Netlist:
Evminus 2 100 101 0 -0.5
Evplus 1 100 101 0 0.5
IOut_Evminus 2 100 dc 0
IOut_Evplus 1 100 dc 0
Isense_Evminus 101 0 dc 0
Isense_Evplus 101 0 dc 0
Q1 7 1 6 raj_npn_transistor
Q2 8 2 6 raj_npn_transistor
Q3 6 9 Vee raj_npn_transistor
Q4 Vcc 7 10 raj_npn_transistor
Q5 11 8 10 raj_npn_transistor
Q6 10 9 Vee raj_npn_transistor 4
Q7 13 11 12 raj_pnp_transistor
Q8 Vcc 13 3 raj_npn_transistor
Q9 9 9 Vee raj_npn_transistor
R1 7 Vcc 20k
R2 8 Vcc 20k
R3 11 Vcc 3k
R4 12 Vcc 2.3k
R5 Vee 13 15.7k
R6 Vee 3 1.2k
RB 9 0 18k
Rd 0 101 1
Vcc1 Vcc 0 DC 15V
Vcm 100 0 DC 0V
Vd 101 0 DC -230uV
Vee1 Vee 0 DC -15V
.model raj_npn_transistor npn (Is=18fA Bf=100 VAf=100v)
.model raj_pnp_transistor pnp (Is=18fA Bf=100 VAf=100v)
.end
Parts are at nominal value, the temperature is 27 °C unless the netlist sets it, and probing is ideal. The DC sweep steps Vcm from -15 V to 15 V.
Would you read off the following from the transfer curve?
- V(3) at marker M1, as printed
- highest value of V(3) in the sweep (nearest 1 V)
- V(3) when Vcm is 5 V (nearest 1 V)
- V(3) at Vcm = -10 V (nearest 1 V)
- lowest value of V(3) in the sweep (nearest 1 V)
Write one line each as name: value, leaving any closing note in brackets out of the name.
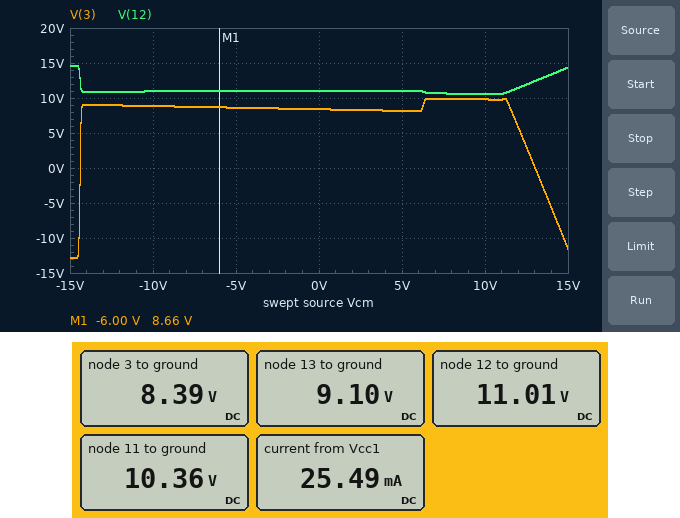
V(3) at marker M1, as printed: 8.66 V
highest value of V(3) in the sweep: 10 V
V(3) when Vcm is 5 V: 8 V
V(3) at Vcm = -10 V: 9 V
lowest value of V(3) in the sweep: -13 V
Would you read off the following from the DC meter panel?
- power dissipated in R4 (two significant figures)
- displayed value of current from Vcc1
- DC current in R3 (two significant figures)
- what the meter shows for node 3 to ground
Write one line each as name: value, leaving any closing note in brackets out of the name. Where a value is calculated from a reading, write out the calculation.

power dissipated in R4: (15 V - 11.01 V)^2 / 2.3 kΩ = 6.9 mW
displayed value of current from Vcc1: 25.49 mA
DC current in R3: (15 V - 10.36 V) / 3 kΩ = 1.5 mA
what the meter shows for node 3 to ground: 8.39 V
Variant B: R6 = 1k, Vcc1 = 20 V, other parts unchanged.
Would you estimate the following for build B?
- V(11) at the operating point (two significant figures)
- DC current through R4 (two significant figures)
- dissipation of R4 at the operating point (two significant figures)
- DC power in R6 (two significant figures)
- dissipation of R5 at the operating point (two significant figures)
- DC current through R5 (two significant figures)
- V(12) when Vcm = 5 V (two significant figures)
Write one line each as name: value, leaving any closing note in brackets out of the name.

V(11) at the operating point: 15 V
DC current through R4: 1.8 mA
dissipation of R4 at the operating point: 7.7 mW
DC power in R6: 590 mW
dissipation of R5 at the operating point: 40 mW
DC current through R5: 1.6 mA
V(12) when Vcm = 5 V: 16 V
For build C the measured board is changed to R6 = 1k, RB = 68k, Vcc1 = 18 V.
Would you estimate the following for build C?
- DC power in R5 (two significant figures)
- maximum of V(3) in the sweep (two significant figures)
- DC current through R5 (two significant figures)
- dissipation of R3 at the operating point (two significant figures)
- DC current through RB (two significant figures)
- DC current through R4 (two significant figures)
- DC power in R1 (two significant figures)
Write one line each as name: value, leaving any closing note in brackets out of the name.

DC power in R5: 1.5 mW
maximum of V(3) in the sweep: -11 V
DC current through R5: 310 µA
dissipation of R3 at the operating point: 650 µW
DC current through RB: 210 µA
DC current through R4: 340 µA
DC power in R1: 280 µW
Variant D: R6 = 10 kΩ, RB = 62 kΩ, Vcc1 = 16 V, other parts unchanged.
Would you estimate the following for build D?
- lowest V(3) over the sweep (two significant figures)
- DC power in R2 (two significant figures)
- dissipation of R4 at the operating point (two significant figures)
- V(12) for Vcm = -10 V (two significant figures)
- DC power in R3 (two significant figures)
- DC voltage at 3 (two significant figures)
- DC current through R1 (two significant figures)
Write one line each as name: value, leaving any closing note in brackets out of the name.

lowest V(3) over the sweep: -15 V
DC power in R2: 330 µW
dissipation of R4 at the operating point: 340 µW
V(12) for Vcm = -10 V: 15 V
DC power in R3: 750 µW
DC voltage at 3: -9.7 V
DC current through R1: 130 µA
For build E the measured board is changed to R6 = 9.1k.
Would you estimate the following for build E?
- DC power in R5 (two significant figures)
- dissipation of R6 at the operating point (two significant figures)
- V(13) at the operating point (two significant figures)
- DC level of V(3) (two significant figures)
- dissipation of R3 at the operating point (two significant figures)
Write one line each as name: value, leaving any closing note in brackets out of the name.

DC power in R5: 43 mW
dissipation of R6 at the operating point: 70 mW
V(13) at the operating point: 11 V
DC level of V(3): 10 V
dissipation of R3 at the operating point: 7.0 mW
